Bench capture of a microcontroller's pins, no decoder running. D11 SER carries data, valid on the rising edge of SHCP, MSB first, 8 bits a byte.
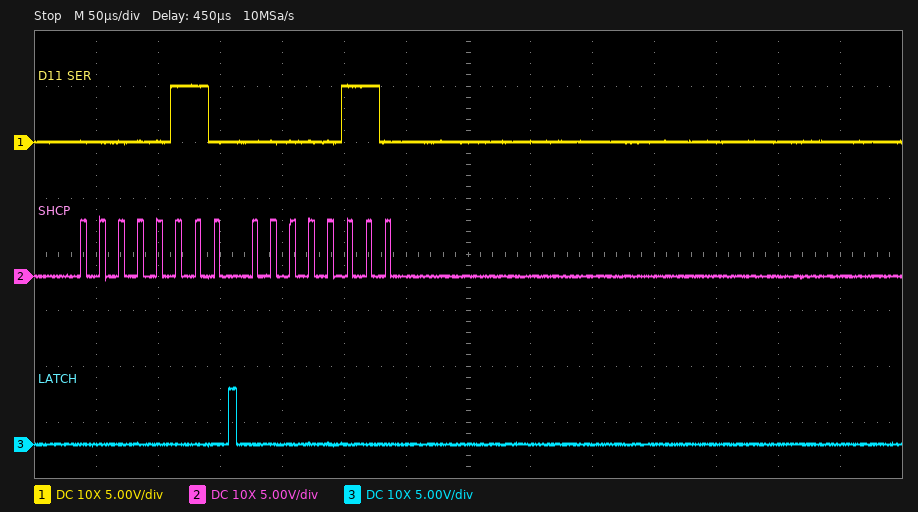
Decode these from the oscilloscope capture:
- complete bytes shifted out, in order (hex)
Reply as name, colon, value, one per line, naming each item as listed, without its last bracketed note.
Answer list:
complete bytes shifted out, in order: 0x06 0x06
